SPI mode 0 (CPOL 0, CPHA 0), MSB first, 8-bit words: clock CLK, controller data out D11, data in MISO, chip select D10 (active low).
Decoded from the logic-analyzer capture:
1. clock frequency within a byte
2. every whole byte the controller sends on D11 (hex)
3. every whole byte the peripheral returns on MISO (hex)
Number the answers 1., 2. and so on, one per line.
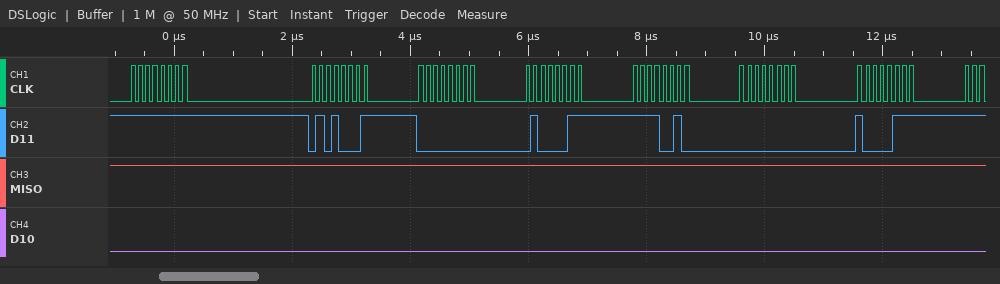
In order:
1. 8 MHz
2. FF 51 00 43 F2 00 87
3. FF FF FF FF FF FF FF
